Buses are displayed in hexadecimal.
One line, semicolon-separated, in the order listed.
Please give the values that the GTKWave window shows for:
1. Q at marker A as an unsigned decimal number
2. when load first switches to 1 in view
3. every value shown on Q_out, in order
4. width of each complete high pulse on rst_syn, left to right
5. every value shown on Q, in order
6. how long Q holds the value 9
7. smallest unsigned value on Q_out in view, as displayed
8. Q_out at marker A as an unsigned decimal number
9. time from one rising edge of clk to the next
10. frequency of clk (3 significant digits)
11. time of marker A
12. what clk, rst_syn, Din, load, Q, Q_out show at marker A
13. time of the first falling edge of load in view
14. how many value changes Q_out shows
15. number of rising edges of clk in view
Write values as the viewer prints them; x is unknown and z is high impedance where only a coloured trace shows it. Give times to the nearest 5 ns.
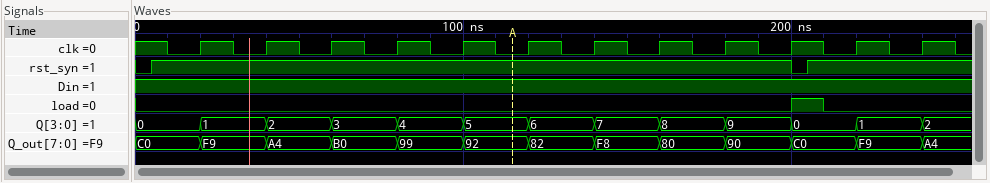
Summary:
5; 200 ns; C0, F9, A4, B0, 99, 92, 82, F8, 80, 90, C0, F9, A4; 195 ns; 0, 1, 2, 3, 4, 5, 6, 7, 8, 9, 0, 1, 2; 20 ns; 80; 146; 20 ns; 50.0 MHz; 115 ns; clk=0, rst_syn=1, Din=1, load=0, Q=5, Q_out=92; 210 ns; 12; 12
